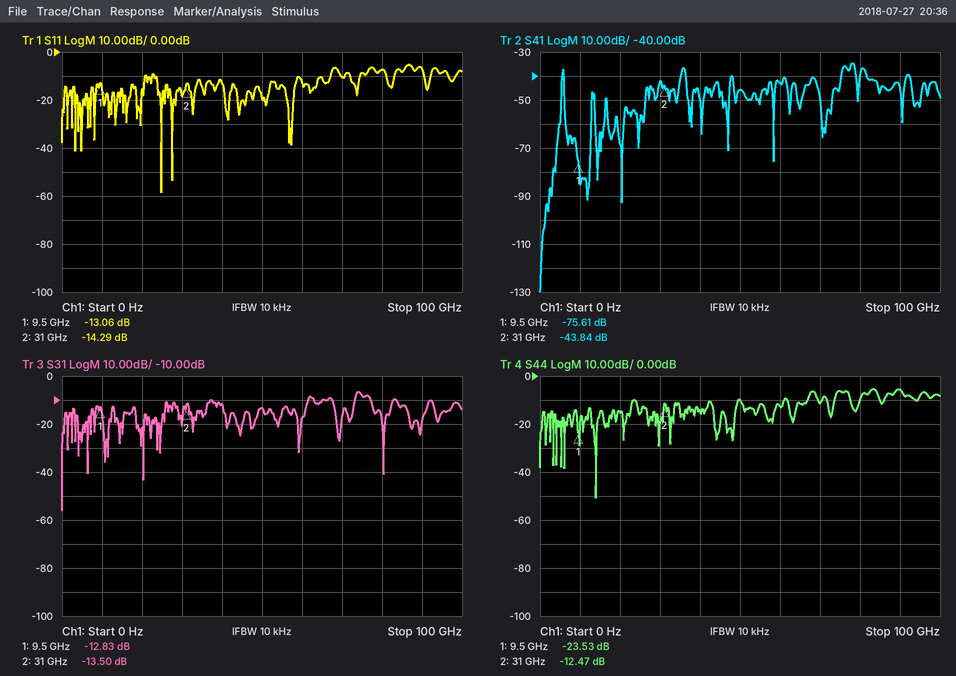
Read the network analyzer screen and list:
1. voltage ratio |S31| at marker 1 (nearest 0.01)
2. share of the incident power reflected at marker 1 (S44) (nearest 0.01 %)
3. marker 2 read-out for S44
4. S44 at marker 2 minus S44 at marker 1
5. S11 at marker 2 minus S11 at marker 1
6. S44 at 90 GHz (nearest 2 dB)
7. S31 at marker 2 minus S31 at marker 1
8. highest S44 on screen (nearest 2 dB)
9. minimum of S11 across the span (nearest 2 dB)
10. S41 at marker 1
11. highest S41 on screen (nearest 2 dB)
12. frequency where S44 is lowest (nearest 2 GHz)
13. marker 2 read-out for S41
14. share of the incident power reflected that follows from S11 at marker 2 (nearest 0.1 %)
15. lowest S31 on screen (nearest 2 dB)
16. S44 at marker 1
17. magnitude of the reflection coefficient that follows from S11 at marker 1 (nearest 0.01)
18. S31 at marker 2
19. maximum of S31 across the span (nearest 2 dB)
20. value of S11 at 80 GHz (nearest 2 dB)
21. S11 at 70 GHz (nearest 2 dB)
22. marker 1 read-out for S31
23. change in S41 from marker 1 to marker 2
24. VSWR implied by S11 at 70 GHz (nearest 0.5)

0.23
0.44 %
-12.47 dB
11.06 dB
-1.23 dB
-6 dB
-0.67 dB
-6 dB
-58 dB
-75.61 dB
-34 dB
14 GHz
-43.84 dB
3.7 %
-56 dB
-23.53 dB
0.22
-13.50 dB
-6 dB
-8 dB
-10 dB
-12.83 dB
31.77 dB
2.0
